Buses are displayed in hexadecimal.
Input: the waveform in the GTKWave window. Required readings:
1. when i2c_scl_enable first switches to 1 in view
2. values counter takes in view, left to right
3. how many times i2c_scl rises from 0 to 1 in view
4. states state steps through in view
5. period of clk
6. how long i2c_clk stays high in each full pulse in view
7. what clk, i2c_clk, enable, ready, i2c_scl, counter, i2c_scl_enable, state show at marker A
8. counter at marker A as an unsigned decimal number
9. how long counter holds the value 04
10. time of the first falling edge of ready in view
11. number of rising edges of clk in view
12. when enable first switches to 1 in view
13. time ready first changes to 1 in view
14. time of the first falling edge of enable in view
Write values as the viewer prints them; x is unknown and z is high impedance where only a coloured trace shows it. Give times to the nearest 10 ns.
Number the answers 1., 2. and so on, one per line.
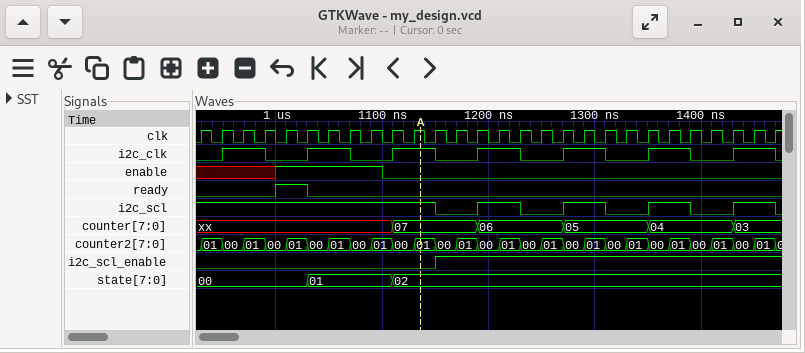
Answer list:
1. 1150 ns
2. xx, 07, 06, 05, 04, 03
3. 4
4. 00, 01, 02
5. 20 ns
6. 40 ns, 40 ns, 40 ns, 40 ns, 40 ns, 40 ns, 40 ns
7. clk=1, i2c_clk=1, enable=0, ready=0, i2c_scl=1, counter=07, i2c_scl_enable=0, state=02
8. 7
9. 80 ns
10. 1030 ns
11. 28
12. 1000 ns
13. 1000 ns
14. 1100 ns
